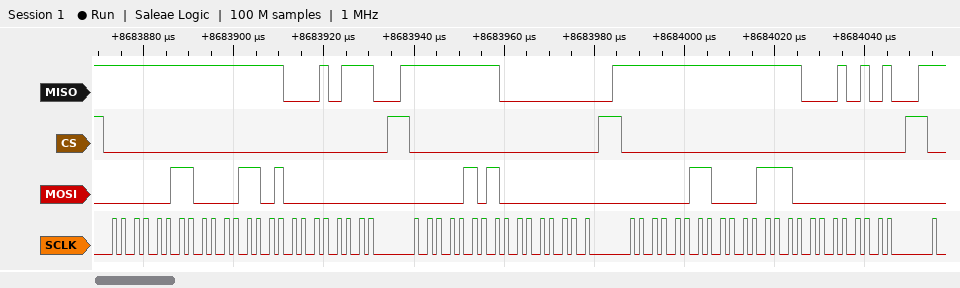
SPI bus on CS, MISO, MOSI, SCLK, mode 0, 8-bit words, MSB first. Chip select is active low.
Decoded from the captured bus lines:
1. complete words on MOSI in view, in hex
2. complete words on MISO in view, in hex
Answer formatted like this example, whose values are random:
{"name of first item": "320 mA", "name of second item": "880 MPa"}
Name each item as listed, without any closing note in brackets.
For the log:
{"complete words on MOSI in view, in hex": "03, 0D, 00, 05, 00, 03, 0E, 00", "complete words on MISO in view, in hex": "FF, FF, 17, FF, 00, FF, FF, 15"}
